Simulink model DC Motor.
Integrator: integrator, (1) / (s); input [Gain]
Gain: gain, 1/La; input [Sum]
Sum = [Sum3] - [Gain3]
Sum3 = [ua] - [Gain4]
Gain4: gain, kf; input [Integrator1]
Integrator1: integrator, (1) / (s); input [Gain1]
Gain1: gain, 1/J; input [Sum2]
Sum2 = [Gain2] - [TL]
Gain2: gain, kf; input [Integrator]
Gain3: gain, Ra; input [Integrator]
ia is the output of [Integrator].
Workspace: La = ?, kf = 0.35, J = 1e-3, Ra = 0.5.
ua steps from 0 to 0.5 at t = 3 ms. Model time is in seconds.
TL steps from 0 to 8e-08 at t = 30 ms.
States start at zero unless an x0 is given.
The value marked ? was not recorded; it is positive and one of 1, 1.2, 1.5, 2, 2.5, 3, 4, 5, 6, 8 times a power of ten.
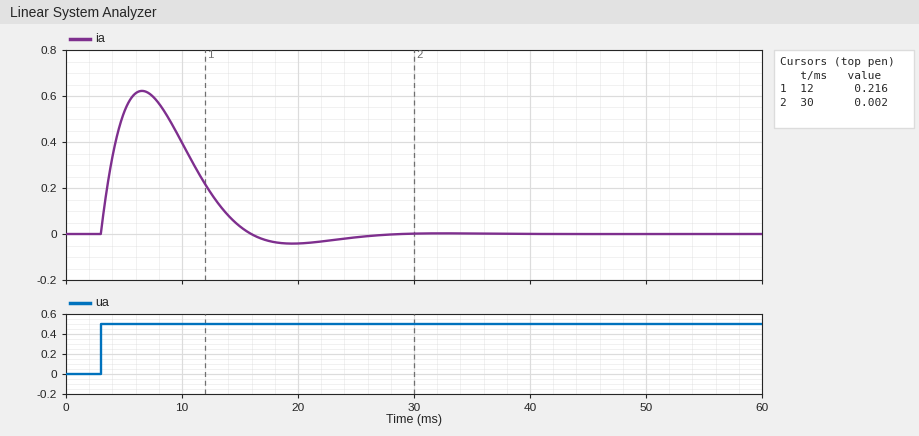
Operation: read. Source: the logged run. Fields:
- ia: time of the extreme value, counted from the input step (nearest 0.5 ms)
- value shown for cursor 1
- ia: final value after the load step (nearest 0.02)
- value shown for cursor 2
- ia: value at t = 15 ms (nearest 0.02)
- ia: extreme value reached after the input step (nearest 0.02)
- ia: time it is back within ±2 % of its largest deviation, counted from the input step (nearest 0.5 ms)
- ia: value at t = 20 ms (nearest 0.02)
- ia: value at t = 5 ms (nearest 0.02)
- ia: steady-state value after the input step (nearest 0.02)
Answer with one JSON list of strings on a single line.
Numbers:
["3.5 ms", "0.216", "0.00", "0.002", "0.04", "0.62", "22.5 ms", "-0.04", "0.52", "0.00"]
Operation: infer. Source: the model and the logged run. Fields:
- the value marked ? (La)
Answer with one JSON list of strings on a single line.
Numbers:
["0.0012"]
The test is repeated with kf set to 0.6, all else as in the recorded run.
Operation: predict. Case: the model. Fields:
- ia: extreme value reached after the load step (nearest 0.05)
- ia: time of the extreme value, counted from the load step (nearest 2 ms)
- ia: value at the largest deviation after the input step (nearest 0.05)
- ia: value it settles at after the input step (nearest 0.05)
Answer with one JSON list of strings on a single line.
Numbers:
["0.00", "6 ms", "0.45", "0.00"]
